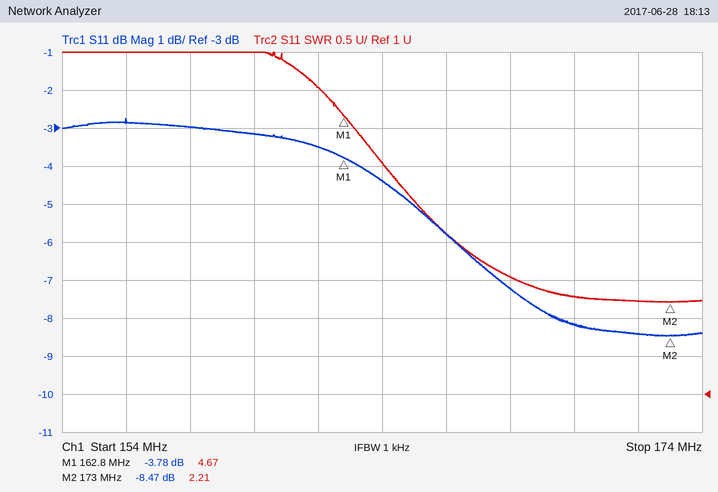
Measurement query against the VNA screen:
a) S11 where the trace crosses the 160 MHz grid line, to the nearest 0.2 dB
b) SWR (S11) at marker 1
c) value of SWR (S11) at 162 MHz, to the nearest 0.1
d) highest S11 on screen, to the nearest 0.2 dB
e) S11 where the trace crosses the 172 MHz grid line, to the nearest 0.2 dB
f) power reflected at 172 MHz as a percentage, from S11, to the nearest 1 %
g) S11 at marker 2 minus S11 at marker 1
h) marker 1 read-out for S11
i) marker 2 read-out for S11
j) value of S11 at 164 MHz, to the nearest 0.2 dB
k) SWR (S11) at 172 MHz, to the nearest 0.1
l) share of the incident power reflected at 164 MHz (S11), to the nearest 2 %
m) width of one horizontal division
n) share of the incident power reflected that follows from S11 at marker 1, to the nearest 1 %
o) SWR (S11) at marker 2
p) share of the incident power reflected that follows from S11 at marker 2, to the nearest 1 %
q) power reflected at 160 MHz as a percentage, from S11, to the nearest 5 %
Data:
-3.2 dB
4.67
5.0
-2.8 dB
-8.4 dB
14 %
-4.69 dB
-3.78 dB
-8.47 dB
-4.4 dB
2.2
36 %
2 MHz
42 %
2.21
14 %
50 %
